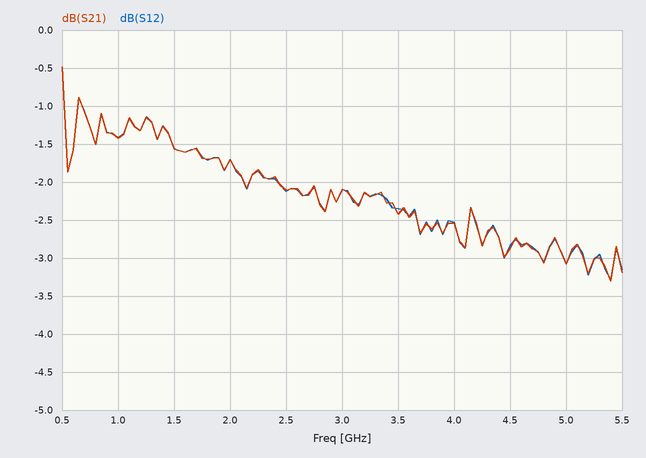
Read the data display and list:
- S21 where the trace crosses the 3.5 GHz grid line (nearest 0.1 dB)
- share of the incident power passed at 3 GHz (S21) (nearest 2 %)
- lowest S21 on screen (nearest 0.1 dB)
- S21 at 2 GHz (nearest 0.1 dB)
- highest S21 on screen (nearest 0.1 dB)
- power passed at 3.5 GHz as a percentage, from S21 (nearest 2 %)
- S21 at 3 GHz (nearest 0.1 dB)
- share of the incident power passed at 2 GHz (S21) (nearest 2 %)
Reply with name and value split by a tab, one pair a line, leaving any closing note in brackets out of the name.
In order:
S21 where the trace crosses the 3.5 GHz grid line	-2.4 dB
share of the incident power passed at 3 GHz (S21)	62 %
lowest S21 on screen	-3.3 dB
S21 at 2 GHz	-1.7 dB
highest S21 on screen	-0.5 dB
power passed at 3.5 GHz as a percentage, from S21	58 %
S21 at 3 GHz	-2.1 dB
share of the incident power passed at 2 GHz (S21)	68 %
